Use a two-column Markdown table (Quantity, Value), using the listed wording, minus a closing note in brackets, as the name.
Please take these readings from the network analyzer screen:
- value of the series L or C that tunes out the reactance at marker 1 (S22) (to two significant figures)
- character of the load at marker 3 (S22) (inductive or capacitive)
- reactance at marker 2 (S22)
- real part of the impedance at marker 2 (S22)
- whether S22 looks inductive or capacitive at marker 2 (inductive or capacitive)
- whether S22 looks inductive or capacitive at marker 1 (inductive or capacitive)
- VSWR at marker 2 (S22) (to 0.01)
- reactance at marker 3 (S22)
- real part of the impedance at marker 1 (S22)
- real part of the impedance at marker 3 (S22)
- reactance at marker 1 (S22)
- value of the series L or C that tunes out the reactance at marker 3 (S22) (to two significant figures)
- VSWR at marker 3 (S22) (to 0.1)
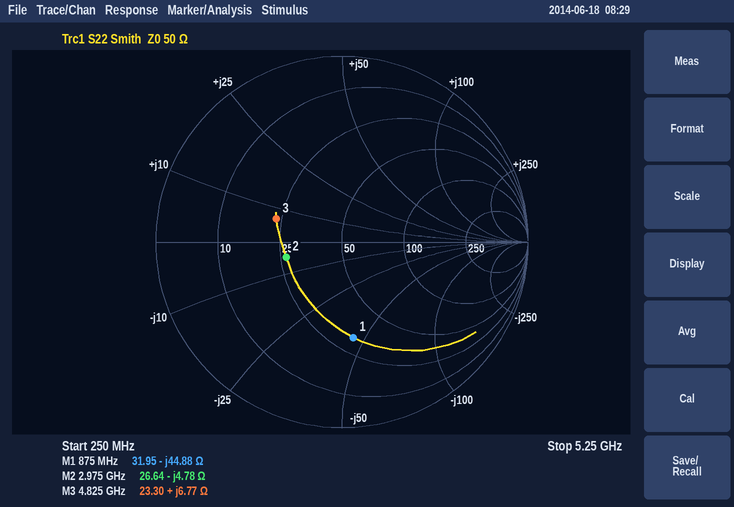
| Quantity | Value |
|---|---|
| value of the series L or C that tunes out the reactance at marker 1 (S22) | 8.2 nH |
| character of the load at marker 3 (S22) | inductive |
| reactance at marker 2 | -4.78 Ω |
| real part of the impedance at marker 2 | 26.64 Ω |
| whether S22 looks inductive or capacitive at marker 2 | capacitive |
| whether S22 looks inductive or capacitive at marker 1 | capacitive |
| VSWR at marker 2 (S22) | 1.90 |
| reactance at marker 3 | +6.77 Ω |
| real part of the impedance at marker 1 | 31.95 Ω |
| real part of the impedance at marker 3 | 23.30 Ω |
| reactance at marker 1 | -44.88 Ω |
| value of the series L or C that tunes out the reactance at marker 3 (S22) | 4.9 pF |
| VSWR at marker 3 (S22) | 2.2 |
